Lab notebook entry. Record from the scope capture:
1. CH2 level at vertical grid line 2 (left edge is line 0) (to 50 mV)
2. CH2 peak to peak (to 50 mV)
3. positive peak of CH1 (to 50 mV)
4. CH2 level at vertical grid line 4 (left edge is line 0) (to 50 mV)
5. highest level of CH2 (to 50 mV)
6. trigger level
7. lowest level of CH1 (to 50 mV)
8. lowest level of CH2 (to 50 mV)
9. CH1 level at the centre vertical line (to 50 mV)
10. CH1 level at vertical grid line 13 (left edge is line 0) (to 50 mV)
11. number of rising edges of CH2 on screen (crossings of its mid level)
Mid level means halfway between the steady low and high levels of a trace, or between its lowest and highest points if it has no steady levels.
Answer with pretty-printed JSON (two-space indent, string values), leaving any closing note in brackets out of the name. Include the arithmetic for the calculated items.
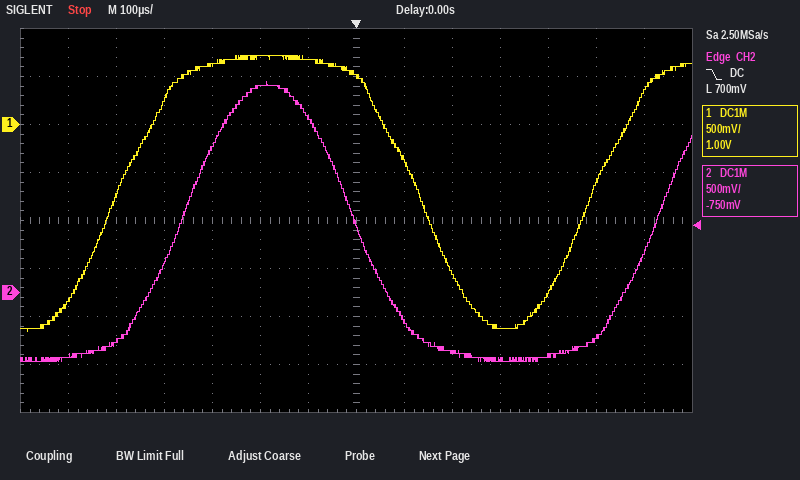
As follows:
{
  "CH2 level at vertical grid line 2 (left edge is line 0)": "-500 mV",
  "CH2 peak to peak": "2.20 V − (-700 mV) = 2.90 V",
  "positive peak of CH1": "700 mV",
  "CH2 level at vertical grid line 4 (left edge is line 0)": "1.50 V",
  "highest level of CH2": "2.20 V",
  "trigger level": "700 mV",
  "lowest level of CH1": "-2.15 V",
  "lowest level of CH2": "-700 mV",
  "CH1 level at the centre vertical line": "500 mV",
  "CH1 level at vertical grid line 13 (left edge is line 0)": "350 mV",
  "number of rising edges of CH2 on screen": "2"
}
